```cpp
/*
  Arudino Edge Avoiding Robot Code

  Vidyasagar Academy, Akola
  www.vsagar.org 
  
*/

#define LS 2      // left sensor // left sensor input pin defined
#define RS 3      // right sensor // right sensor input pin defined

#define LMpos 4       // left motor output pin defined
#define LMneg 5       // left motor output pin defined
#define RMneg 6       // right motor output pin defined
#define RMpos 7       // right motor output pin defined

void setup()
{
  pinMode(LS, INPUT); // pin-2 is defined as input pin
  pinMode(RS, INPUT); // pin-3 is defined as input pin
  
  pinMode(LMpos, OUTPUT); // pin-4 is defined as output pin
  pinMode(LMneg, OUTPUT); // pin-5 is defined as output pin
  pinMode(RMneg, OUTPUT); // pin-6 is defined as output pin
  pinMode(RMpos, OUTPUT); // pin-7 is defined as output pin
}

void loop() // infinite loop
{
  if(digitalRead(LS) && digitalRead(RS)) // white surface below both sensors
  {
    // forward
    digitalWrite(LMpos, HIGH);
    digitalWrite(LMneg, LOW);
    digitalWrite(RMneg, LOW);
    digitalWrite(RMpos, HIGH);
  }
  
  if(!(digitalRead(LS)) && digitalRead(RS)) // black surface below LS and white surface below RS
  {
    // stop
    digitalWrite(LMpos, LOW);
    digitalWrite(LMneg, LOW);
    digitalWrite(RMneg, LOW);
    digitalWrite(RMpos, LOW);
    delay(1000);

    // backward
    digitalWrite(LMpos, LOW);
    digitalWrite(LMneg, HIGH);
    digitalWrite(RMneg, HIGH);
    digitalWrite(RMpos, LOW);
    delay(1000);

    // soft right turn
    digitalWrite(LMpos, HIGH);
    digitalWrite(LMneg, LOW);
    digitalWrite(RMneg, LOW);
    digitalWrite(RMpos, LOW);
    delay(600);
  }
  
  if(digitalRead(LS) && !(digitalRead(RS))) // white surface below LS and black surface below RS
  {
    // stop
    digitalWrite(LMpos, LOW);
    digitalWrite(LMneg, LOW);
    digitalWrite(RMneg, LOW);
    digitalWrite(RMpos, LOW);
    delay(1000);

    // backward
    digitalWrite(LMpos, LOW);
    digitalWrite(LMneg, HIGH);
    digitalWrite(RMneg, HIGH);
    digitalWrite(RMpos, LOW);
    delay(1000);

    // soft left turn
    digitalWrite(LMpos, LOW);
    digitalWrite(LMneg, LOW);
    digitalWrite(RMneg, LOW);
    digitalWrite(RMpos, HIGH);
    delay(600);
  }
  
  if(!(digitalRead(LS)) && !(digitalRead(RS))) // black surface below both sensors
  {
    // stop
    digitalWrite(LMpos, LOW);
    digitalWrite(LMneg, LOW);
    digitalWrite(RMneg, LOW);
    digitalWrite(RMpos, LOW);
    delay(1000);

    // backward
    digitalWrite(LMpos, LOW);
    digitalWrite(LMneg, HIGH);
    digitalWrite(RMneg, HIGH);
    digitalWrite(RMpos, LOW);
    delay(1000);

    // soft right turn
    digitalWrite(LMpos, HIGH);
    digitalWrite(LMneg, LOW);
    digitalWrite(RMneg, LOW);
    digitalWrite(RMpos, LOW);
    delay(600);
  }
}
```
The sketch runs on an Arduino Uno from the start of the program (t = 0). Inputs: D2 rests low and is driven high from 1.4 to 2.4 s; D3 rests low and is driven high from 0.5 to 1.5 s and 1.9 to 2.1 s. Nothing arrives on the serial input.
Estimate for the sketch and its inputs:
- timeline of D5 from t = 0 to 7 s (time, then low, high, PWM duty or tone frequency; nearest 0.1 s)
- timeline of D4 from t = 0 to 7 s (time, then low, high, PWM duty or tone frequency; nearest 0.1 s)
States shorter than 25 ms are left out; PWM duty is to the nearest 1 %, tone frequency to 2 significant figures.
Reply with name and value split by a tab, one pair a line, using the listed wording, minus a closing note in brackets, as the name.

timeline of D5 from t = 0 to 7 s	0 s low; 1 s high; 2 s low; 3.6 s high; 4.6 s low; 6.2 s high
timeline of D4 from t = 0 to 7 s	0 s low; 2 s high; 2.6 s low; 4.6 s high; 5.2 s low
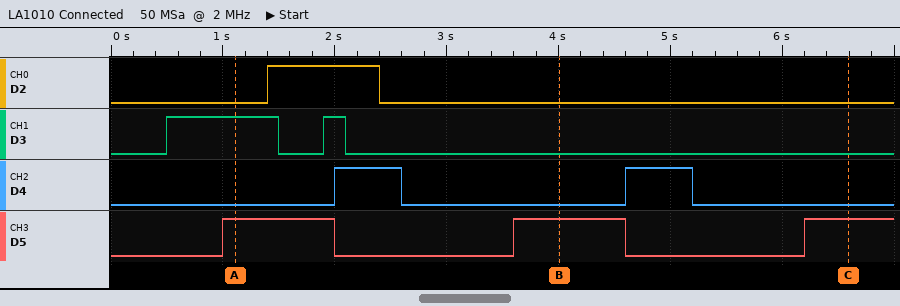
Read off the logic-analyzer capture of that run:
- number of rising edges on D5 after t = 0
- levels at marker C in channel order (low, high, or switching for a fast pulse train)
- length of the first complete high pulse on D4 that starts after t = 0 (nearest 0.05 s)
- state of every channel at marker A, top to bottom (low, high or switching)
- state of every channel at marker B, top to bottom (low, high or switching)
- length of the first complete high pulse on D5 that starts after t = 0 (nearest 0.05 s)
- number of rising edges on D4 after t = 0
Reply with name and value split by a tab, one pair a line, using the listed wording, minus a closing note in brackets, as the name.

number of rising edges on D5 after t = 0	3
levels at marker C in channel order	D2 low, D3 low, D4 low, D5 high
length of the first complete high pulse on D4 that starts after t = 0	0.60 s
state of every channel at marker A, top to bottom	D2 low, D3 high, D4 low, D5 high
state of every channel at marker B, top to bottom	D2 low, D3 low, D4 low, D5 high
length of the first complete high pulse on D5 that starts after t = 0	1.00 s
number of rising edges on D4 after t = 0	2
